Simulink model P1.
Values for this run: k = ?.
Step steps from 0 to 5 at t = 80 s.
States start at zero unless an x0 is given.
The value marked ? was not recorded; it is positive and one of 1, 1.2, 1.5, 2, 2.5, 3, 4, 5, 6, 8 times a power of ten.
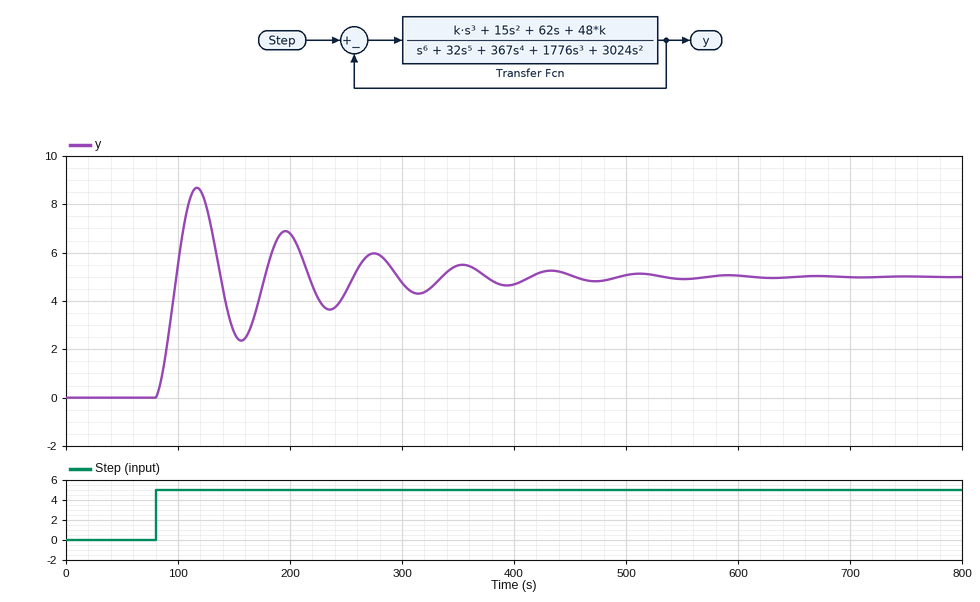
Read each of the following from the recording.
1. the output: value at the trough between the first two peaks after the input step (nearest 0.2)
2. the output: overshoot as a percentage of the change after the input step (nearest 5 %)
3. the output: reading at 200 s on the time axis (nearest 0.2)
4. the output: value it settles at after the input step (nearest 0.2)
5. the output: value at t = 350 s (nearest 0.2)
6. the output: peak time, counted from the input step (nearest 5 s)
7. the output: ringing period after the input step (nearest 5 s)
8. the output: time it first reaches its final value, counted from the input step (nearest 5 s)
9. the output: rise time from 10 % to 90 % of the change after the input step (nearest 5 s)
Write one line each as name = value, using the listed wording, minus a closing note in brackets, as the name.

the output: value at the trough between the first two peaks after the input step = 2.4
the output: overshoot as a percentage of the change after the input step = 75 %
the output: reading at 200 s on the time axis = 6.8
the output: value it settles at after the input step = 5.0
the output: value at t = 350 s = 5.4
the output: peak time, counted from the input step = 35 s
the output: ringing period after the input step = 80 s
the output: time it first reaches its final value, counted from the input step = 20 s
the output: rise time from 10 % to 90 % of the change after the input step = 15 s
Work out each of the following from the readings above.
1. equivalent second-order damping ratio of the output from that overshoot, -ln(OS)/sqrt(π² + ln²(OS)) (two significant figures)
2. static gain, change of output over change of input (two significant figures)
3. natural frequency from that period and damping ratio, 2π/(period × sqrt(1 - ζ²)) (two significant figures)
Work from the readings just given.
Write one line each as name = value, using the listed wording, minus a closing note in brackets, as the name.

equivalent second-order damping ratio of the output from that overshoot, -ln(OS)/sqrt(π² + ln²(OS)) = 0.091
static gain, change of output over change of input = 1.0
natural frequency from that period and damping ratio, 2π/(period × sqrt(1 - ζ²)) = 0.079 rad/s
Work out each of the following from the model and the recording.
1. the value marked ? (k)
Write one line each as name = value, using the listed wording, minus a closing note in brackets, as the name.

the value marked ? = 0.4
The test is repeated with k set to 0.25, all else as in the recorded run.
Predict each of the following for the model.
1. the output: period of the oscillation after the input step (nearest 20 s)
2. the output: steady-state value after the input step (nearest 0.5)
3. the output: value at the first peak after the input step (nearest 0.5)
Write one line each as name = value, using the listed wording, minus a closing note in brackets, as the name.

the output: period of the oscillation after the input step = 100 s
the output: steady-state value after the input step = 5.0
the output: value at the first peak after the input step = 8.5
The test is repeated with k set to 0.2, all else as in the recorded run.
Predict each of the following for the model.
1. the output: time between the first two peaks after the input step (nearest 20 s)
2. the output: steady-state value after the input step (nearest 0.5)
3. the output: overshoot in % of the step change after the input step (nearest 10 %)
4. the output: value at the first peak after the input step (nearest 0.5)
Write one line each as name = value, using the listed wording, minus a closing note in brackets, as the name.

the output: time between the first two peaks after the input step = 120 s
the output: steady-state value after the input step = 5.0
the output: overshoot in % of the step change after the input step = 60 %
the output: value at the first peak after the input step = 8.0
